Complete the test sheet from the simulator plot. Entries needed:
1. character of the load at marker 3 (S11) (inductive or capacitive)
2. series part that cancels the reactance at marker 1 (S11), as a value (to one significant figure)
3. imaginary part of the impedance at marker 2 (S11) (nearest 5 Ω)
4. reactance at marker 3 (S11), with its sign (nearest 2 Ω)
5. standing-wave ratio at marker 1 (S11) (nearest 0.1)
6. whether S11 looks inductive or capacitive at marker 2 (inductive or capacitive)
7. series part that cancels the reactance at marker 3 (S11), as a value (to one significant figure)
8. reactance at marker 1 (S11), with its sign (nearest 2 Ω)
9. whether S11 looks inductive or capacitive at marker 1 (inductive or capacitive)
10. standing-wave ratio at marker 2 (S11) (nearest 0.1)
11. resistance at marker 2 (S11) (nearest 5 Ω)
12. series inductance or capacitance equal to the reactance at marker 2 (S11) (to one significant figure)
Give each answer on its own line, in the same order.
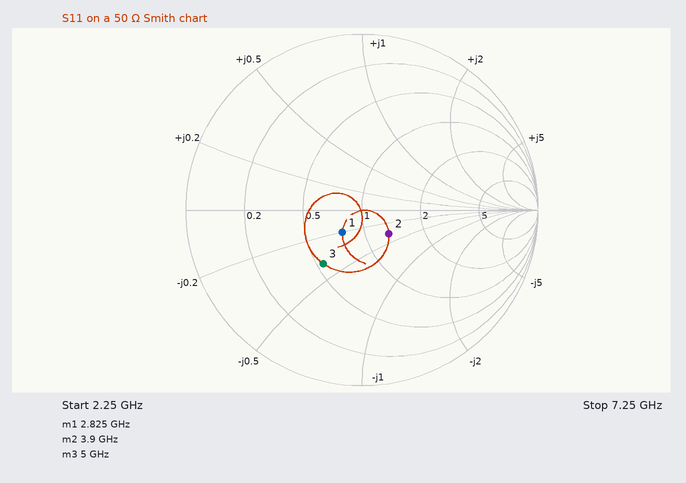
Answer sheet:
capacitive
600 pH
-20 Ω
-20 Ω
1.4
capacitive
600 pH
-10 Ω
capacitive
1.5
65 Ω
2 pF
